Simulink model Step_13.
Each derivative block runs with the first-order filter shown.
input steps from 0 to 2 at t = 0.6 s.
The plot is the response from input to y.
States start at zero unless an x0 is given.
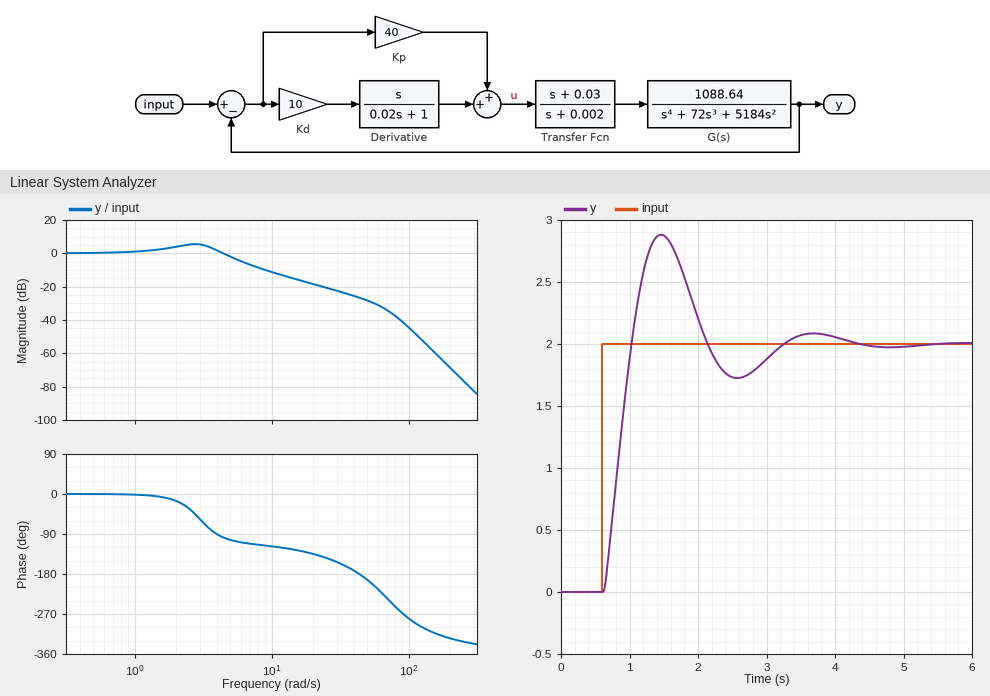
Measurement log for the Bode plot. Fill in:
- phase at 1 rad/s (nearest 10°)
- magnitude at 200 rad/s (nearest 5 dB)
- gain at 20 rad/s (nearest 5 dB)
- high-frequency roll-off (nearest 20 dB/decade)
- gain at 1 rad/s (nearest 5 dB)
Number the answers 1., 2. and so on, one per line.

1. 0°
2. -70 dB
3. -20 dB
4. -80 dB/decade
5. 0 dB
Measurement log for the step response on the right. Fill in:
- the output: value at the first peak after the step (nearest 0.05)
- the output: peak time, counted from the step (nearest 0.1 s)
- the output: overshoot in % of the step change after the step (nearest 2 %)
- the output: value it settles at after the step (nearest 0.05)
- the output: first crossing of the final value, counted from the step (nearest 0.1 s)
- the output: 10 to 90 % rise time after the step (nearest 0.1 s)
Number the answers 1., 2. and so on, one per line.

1. 2.90
2. 0.9 s
3. 44 %
4. 2.00
5. 0.4 s
6. 0.3 s
